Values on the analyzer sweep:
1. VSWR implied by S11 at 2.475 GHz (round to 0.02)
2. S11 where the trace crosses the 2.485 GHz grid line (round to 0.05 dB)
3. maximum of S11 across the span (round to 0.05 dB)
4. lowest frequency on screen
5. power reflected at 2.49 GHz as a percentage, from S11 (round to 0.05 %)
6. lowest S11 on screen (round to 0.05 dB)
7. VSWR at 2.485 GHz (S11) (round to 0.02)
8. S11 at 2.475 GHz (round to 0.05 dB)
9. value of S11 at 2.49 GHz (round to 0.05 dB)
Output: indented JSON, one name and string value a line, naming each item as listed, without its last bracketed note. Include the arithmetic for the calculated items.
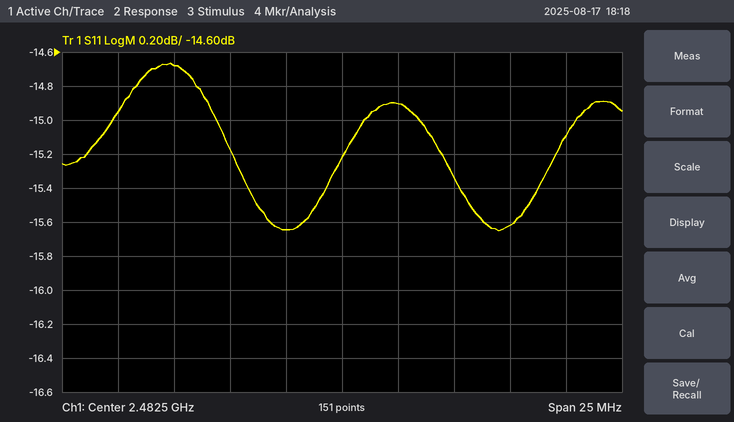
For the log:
{
  "VSWR implied by S11 at 2.475 GHz": "|Γ| = 10^(-14.7/20) = 0.1841; VSWR = (1 + 0.1841)/(1 − 0.1841) ≈ 1.45, so 1.46 to the nearest 0.02",
  "S11 where the trace crosses the 2.485 GHz grid line": "-14.90 dB",
  "maximum of S11 across the span": "-14.65 dB",
  "lowest frequency on screen": "2.47 GHz",
  "power reflected at 2.49 GHz as a percentage, from S11": "10^(-15.6/10) ≈ 2.75 %",
  "lowest S11 on screen": "-15.65 dB",
  "VSWR at 2.485 GHz (S11)": "|Γ| = 10^(-14.9/20) = 0.1799; VSWR = (1 + 0.1799)/(1 − 0.1799) ≈ 1.44",
  "S11 at 2.475 GHz": "-14.70 dB",
  "value of S11 at 2.49 GHz": "-15.60 dB"
}
